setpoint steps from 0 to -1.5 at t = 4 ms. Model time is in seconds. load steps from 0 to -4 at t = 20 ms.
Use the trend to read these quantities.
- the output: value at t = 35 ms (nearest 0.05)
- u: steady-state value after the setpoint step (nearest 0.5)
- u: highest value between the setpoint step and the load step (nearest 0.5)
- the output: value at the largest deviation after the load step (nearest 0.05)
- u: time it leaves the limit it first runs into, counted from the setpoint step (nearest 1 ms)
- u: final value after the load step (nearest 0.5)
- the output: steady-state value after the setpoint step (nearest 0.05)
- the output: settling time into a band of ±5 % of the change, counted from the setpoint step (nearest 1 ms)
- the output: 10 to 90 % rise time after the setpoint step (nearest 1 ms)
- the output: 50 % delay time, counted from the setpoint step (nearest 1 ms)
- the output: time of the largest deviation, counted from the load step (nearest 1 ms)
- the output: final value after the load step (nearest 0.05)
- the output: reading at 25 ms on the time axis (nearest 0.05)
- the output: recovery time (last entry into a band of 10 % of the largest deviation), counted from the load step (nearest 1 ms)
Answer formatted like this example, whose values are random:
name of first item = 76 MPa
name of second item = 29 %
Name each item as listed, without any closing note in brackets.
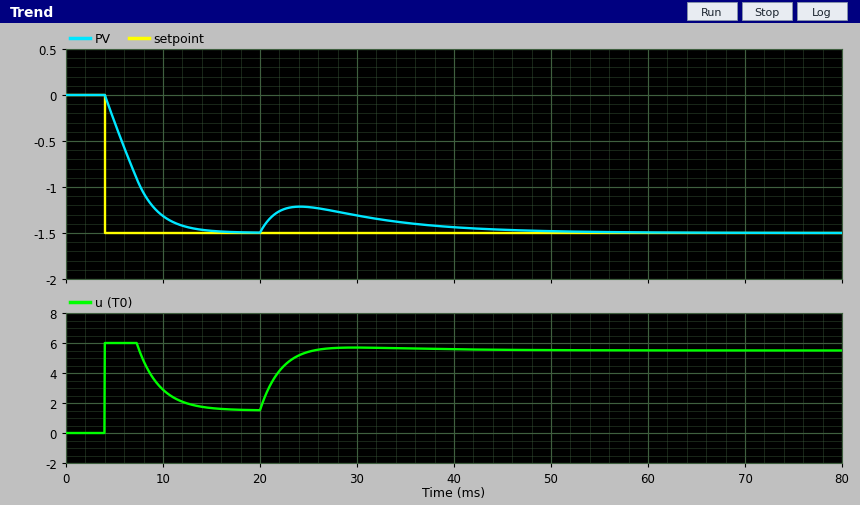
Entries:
the output: value at t = 35 ms = -1.40
u: steady-state value after the setpoint step = 1.5
u: highest value between the setpoint step and the load step = 6.0
the output: value at the largest deviation after the load step = -1.20
u: time it leaves the limit it first runs into, counted from the setpoint step = 3 ms
u: final value after the load step = 5.5
the output: steady-state value after the setpoint step = -1.50
the output: settling time into a band of ±5 % of the change, counted from the setpoint step = 8 ms
the output: 10 to 90 % rise time after the setpoint step = 6 ms
the output: 50 % delay time, counted from the setpoint step = 3 ms
the output: time of the largest deviation, counted from the load step = 4 ms
the output: final value after the load step = -1.50
the output: reading at 25 ms on the time axis = -1.20
the output: recovery time (last entry into a band of 10 % of the largest deviation), counted from the load step = 27 ms
